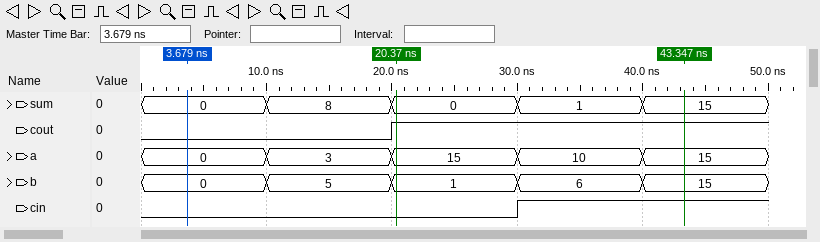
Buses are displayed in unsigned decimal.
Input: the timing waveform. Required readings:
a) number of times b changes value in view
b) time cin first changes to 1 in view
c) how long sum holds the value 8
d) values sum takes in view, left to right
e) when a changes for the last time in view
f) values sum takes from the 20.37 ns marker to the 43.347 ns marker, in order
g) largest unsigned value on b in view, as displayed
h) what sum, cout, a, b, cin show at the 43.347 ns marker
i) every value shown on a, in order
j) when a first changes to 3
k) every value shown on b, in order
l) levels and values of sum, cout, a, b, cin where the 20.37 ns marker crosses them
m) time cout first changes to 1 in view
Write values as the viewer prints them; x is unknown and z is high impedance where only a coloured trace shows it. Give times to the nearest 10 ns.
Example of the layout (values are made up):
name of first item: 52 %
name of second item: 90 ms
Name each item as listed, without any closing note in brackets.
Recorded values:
number of times b changes value in view: 4
time cin first changes to 1 in view: 30 ns
how long sum holds the value 8: 10 ns
values sum takes in view, left to right: 0, 8, 0, 1, 15
when a changes for the last time in view: 40 ns
values sum takes from the 20.37 ns marker to the 43.347 ns marker, in order: 0, 1, 15
largest unsigned value on b in view, as displayed: 15
what sum, cout, a, b, cin show at the 43.347 ns marker: sum=15, cout=1, a=15, b=15, cin=1
every value shown on a, in order: 0, 3, 15, 10, 15
when a first changes to 3: 10 ns
every value shown on b, in order: 0, 5, 1, 6, 15
levels and values of sum, cout, a, b, cin where the 20.37 ns marker crosses them: sum=0, cout=1, a=15, b=1, cin=0
time cout first changes to 1 in view: 20 ns
